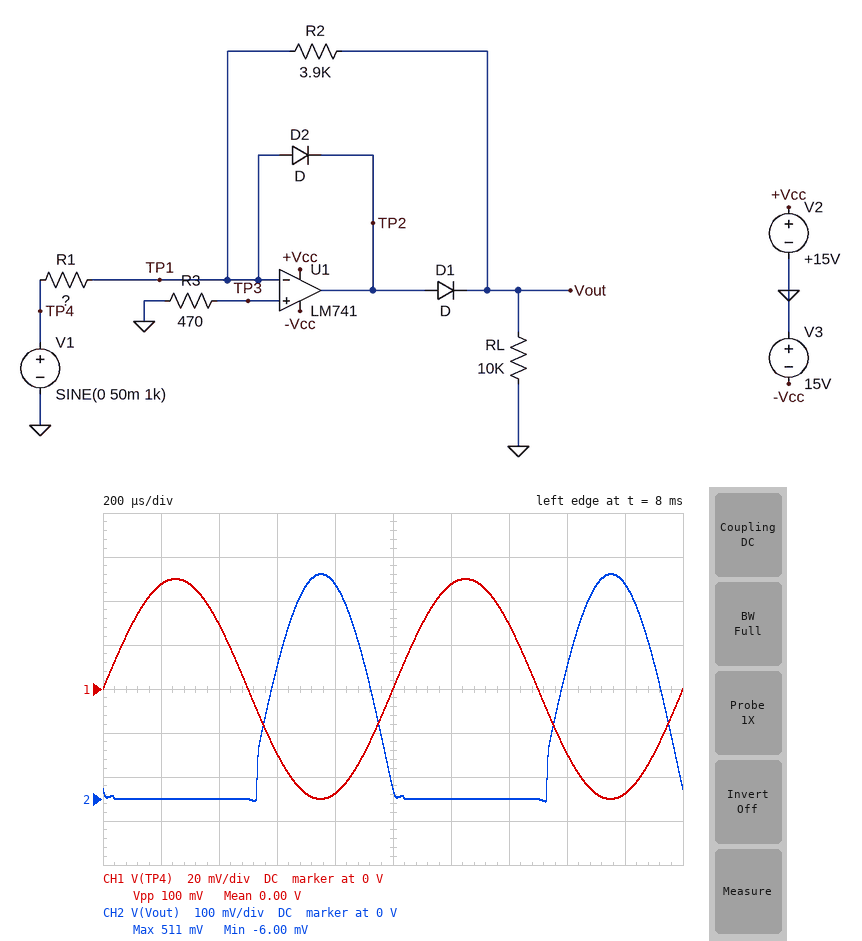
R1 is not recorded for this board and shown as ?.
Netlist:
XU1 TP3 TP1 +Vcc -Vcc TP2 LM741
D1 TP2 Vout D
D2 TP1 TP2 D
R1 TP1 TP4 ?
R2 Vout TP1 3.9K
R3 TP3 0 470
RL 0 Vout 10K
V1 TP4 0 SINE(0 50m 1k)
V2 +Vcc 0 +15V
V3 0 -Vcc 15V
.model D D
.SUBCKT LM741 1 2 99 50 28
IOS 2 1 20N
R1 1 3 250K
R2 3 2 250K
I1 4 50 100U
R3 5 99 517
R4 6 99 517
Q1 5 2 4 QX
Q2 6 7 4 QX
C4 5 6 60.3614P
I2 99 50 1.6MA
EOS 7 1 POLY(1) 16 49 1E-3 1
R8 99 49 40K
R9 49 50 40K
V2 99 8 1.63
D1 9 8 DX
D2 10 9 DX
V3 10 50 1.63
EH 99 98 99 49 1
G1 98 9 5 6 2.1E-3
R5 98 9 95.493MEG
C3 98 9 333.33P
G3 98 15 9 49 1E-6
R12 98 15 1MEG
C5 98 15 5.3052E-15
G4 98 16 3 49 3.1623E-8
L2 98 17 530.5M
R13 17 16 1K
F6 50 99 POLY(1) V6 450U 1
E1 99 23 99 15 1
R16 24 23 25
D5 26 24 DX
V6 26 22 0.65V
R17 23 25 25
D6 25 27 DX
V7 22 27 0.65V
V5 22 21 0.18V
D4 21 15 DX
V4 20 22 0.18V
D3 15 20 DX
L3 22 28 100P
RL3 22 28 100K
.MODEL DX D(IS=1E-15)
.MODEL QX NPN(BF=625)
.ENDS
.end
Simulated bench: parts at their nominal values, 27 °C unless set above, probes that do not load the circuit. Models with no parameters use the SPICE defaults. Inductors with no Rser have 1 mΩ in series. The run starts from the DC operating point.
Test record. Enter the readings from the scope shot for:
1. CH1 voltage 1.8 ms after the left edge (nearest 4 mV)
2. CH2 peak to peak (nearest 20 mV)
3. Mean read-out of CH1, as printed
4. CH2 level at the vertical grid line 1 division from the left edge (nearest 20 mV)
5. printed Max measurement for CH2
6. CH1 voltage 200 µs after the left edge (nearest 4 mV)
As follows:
-48 mV
520 mV
0.00 V
0 V
511 mV
48 mV
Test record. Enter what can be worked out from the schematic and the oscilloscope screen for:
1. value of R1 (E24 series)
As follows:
390 Ω
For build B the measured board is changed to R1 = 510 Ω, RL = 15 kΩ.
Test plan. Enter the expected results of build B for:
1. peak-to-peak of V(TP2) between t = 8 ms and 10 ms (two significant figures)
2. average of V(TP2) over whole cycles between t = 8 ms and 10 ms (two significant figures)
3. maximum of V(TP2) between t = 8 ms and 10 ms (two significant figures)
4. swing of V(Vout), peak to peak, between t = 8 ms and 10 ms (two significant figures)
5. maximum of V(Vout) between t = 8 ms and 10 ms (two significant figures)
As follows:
1.6 V
140 mV
990 mV
400 mV
390 mV
